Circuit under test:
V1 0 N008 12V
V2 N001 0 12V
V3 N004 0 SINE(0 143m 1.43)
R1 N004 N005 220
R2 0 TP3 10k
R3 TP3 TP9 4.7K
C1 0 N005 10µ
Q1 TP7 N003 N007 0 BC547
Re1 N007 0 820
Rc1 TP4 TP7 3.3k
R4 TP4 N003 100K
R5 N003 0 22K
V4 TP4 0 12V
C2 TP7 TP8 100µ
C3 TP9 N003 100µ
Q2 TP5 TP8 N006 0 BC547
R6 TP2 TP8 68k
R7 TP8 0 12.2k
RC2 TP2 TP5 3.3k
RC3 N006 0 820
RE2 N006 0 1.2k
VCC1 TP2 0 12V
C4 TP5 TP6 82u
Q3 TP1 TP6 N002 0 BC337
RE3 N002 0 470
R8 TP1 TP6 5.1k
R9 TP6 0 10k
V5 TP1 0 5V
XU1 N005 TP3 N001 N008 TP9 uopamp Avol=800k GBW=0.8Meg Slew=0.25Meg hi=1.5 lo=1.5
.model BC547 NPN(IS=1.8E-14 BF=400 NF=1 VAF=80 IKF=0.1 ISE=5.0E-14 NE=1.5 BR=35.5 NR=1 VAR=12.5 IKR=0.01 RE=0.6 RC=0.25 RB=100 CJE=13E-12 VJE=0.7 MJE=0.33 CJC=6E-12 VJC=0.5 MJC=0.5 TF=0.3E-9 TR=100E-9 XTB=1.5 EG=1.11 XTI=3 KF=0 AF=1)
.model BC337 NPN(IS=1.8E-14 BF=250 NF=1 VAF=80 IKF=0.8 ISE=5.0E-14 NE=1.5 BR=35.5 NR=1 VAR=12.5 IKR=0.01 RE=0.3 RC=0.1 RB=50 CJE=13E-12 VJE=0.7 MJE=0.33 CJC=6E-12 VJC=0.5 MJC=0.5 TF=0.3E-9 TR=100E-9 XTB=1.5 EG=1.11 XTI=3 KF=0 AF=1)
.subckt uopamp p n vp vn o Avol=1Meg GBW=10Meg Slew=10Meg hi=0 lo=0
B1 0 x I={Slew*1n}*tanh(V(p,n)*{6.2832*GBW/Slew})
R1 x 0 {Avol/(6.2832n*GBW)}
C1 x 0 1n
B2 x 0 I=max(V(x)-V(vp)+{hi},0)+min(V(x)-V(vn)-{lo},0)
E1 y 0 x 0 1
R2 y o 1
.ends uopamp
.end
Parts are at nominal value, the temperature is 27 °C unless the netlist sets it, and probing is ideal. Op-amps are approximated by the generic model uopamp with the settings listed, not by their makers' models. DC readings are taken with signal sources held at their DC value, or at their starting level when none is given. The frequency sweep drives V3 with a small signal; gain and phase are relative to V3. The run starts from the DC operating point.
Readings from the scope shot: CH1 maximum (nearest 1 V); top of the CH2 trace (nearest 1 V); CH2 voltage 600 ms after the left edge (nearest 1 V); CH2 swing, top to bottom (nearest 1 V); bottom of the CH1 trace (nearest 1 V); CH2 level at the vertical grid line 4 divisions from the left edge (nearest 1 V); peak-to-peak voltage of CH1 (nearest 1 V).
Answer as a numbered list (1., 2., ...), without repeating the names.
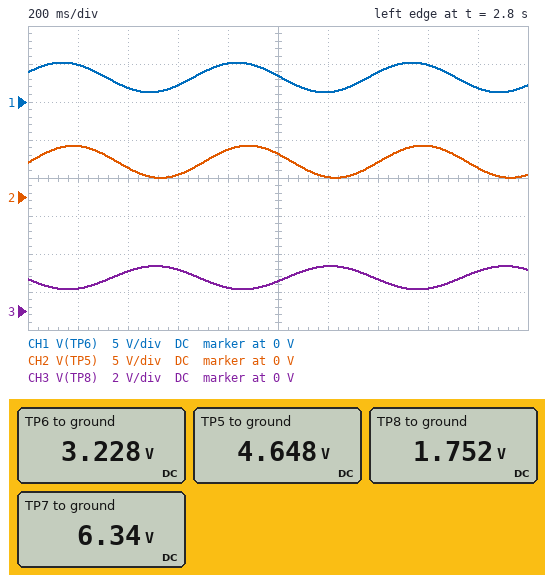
1. 5 V
2. 7 V
3. 3 V
4. 4 V
5. 1 V
6. 6 V
7. 4 V
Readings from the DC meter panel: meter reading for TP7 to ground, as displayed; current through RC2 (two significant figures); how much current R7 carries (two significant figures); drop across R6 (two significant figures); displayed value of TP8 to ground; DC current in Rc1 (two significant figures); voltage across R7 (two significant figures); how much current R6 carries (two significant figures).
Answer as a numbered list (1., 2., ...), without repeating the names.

1. 6.34 V
2. 2.2 mA
3. 140 µA
4. 10 V
5. 1.752 V
6. 1.7 mA
7. 1.8 V
8. 150 µA
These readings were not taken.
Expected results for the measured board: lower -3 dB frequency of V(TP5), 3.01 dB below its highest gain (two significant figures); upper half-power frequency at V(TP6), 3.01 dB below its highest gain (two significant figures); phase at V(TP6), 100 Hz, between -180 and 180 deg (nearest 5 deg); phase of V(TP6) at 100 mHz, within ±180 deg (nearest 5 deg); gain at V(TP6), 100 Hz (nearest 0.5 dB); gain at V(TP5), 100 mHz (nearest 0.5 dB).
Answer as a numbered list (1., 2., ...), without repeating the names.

1. 110 mHz
2. 73 Hz
3. -55 deg
4. 165 deg
5. 18.5 dB
6. 22.0 dB
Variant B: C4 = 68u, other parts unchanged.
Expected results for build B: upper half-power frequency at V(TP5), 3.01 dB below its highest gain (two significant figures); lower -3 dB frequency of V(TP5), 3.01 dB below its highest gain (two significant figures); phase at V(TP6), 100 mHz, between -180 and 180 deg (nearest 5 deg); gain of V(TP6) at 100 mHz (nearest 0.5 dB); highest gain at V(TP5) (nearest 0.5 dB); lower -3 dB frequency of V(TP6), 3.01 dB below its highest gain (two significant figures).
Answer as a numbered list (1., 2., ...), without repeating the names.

1. 2.0 Hz
2. 120 mHz
3. 170 deg
4. 5.0 dB
5. 26.5 dB
6. 410 mHz
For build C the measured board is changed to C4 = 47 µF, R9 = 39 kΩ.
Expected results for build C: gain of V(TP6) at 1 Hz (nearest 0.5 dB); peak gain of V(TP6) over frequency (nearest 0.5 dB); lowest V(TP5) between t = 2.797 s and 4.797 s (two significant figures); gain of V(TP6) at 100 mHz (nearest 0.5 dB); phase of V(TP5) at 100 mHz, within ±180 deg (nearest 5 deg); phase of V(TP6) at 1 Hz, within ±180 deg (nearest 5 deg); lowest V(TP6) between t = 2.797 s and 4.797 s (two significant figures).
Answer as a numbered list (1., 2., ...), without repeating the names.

1. 23.0 dB
2. 24.0 dB
3. 2.2 V
4. 4.0 dB
5. 90 deg
6. 35 deg
7. 2.0 V
